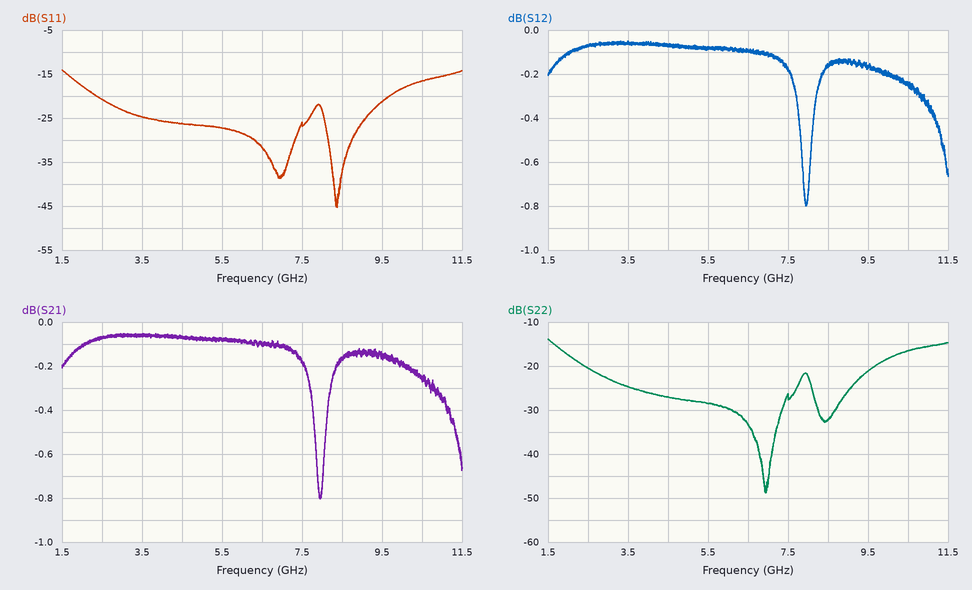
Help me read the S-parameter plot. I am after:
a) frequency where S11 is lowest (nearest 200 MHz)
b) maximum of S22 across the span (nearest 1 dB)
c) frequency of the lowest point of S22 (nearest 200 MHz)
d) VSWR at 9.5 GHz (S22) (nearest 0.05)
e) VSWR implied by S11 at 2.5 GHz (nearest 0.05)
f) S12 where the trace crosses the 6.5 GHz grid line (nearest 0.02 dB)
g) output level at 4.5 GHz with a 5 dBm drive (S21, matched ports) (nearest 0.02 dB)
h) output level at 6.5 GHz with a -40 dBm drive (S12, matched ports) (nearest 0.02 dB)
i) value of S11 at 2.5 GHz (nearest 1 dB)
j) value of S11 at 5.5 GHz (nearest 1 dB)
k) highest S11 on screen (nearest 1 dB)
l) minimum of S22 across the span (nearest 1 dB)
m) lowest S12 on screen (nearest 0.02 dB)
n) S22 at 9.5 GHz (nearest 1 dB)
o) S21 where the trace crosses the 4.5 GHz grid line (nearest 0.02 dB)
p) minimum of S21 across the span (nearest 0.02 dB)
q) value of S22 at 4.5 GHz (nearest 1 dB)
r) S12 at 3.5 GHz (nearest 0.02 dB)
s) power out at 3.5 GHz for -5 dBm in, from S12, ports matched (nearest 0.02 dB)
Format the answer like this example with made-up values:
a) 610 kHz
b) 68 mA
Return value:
a) 8.4 GHz
b) -14 dB
c) 7.0 GHz
d) 1.20
e) 1.20
f) -0.10 dB
g) 4.94 dBm
h) -40.10 dBm
i) -21 dB
j) -27 dB
k) -14 dB
l) -49 dB
m) -0.80 dB
n) -21 dB
o) -0.06 dB
p) -0.80 dB
q) -27 dB
r) -0.06 dB
s) -5.06 dBm
